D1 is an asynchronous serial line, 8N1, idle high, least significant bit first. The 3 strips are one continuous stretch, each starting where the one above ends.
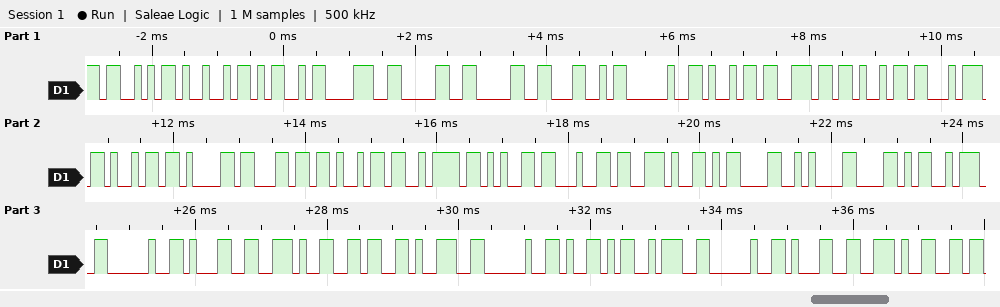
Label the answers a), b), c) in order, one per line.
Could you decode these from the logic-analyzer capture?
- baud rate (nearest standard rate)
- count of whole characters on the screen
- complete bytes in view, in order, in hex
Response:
a) 9600 baud
b) 35
c) 53 49 4D 38 30 30 4C 20 69 6E 69 74 69 61 6C 69 7A 65 64 2E 0D 0A 58 3A 20 31 2E 36 39 20 59 3A 20 31 2E
